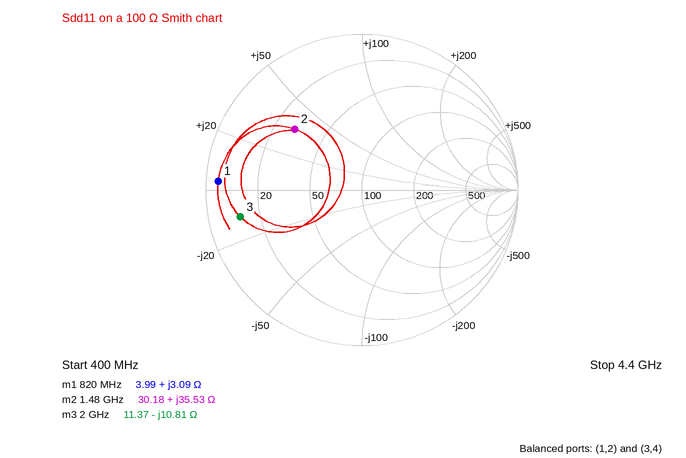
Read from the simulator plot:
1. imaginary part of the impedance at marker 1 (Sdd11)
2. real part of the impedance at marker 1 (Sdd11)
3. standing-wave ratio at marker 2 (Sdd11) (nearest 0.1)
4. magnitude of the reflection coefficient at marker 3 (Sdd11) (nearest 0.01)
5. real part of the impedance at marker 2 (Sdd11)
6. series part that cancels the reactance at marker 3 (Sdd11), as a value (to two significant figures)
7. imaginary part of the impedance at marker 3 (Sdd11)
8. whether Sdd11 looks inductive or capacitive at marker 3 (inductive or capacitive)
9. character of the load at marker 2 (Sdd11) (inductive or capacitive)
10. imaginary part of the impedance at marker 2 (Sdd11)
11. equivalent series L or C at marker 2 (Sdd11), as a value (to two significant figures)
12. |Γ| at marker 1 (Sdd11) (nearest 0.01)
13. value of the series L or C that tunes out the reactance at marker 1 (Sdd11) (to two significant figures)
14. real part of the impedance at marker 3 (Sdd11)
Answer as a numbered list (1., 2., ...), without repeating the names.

1. +3.09 Ω
2. 3.99 Ω
3. 3.8
4. 0.80
5. 30.18 Ω
6. 860 pH
7. -10.81 Ω
8. capacitive
9. inductive
10. +35.53 Ω
11. 3.8 nH
12. 0.92
13. 63 pF
14. 11.37 Ω
